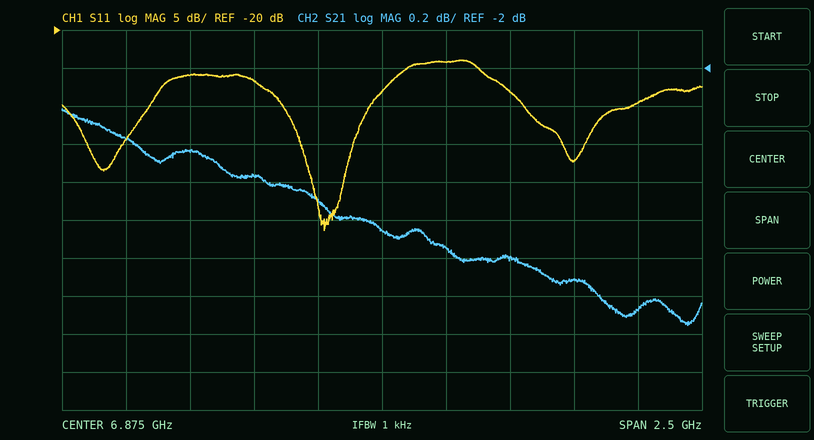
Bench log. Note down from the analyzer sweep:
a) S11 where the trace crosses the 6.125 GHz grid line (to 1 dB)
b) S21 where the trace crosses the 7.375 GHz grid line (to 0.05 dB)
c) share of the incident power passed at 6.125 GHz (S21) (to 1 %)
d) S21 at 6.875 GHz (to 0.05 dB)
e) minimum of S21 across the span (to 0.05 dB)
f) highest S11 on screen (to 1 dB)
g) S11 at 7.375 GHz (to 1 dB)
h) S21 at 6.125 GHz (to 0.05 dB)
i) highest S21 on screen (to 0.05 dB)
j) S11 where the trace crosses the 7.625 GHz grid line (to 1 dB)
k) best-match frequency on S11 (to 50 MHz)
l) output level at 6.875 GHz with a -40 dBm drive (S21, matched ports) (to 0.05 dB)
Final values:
-26 dB
-3.00 dB
57 %
-2.85 dB
-3.35 dB
-24 dB
-28 dB
-2.45 dB
-2.20 dB
-37 dB
6.65 GHz
-42.85 dBm
